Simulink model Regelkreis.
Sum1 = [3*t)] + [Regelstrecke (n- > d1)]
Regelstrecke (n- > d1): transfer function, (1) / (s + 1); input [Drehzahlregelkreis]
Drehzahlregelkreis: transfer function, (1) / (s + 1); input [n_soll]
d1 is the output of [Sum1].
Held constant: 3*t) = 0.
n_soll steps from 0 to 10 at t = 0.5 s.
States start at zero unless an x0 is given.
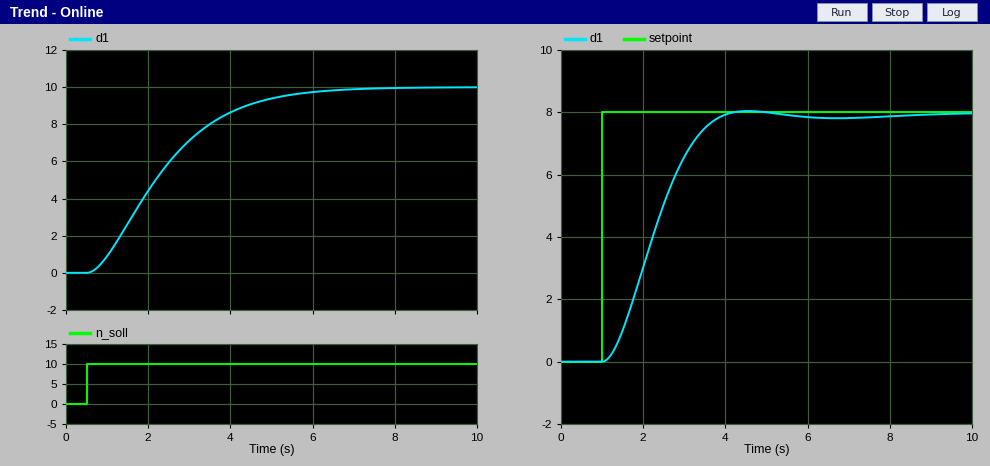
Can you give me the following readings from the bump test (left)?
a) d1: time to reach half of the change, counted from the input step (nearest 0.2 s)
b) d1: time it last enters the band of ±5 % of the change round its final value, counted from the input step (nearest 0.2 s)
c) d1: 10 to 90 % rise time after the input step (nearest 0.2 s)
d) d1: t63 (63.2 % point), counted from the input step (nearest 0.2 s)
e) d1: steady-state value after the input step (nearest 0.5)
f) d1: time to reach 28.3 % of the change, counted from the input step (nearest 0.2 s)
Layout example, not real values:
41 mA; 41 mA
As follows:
1.6 s; 4.8 s; 3.4 s; 2.2 s; 10.0; 1.0 s
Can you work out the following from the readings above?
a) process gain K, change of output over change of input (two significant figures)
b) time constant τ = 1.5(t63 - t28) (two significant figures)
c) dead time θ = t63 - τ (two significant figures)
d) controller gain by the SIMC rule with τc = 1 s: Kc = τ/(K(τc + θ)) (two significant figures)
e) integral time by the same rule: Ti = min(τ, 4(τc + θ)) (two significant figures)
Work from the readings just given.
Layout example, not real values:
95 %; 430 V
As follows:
1.0; 1.8 s; 0.40 s; 1.3; 1.8 s
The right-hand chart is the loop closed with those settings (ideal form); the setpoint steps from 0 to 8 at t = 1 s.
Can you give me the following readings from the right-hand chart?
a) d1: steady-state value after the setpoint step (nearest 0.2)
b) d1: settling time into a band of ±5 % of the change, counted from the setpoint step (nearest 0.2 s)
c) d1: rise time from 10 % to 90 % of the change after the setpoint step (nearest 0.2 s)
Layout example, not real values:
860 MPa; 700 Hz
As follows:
8.0; 2.6 s; 1.8 s
